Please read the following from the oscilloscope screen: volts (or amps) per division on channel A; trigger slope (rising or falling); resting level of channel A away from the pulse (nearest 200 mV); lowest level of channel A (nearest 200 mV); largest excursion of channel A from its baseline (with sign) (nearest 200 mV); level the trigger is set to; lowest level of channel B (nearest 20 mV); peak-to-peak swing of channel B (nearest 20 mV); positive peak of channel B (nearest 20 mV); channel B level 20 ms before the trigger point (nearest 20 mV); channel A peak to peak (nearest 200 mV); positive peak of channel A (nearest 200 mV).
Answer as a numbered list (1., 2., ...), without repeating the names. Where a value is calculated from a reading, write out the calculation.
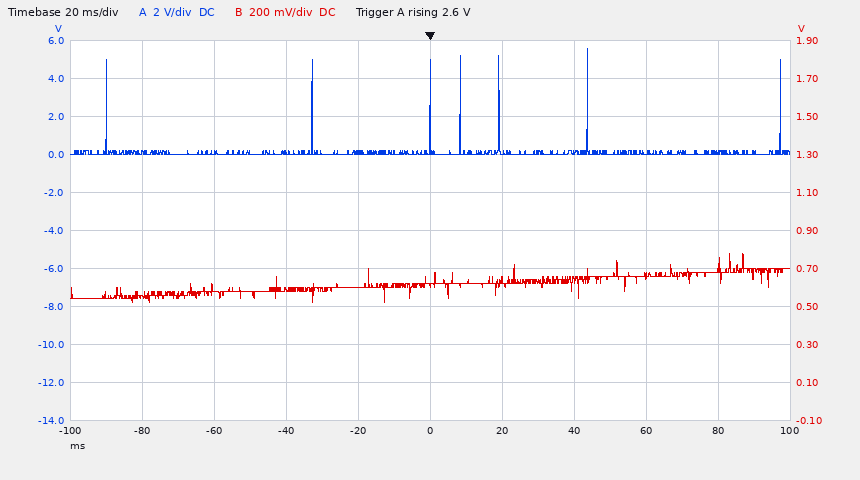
1. 2 V
2. rising
3. 0.0 V
4. 0.0 V
5. 5.6 V − (0.0 V) = +5.6 V
6. 2.6 V
7. 520 mV
8. 780 mV − (520 mV) = 260 mV
9. 780 mV
10. 600 mV
11. 5.6 V − (0.0 V) = 5.6 V
12. 5.6 V
